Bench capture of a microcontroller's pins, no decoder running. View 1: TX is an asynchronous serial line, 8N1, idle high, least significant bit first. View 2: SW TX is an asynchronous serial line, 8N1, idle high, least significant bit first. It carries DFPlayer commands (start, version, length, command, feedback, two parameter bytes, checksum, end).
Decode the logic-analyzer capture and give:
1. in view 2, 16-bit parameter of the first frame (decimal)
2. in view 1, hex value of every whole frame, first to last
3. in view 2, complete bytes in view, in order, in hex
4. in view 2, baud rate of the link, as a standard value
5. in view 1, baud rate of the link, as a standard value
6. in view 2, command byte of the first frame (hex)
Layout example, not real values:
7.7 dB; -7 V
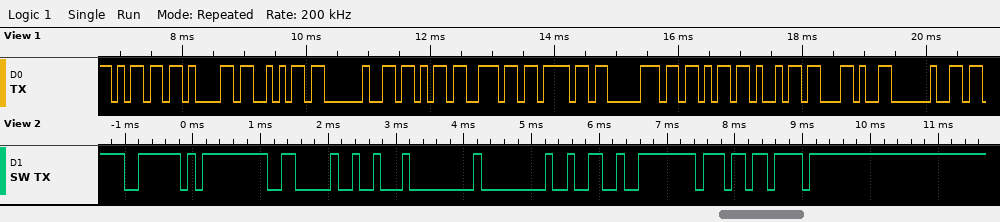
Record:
50; 6D 61 6A 20 6B 6E 6F 70 6B 69 2C 20; 7E FF 06 12 00 00 32 FE B7 EF; 9600 baud; 9600 baud; 0x12
